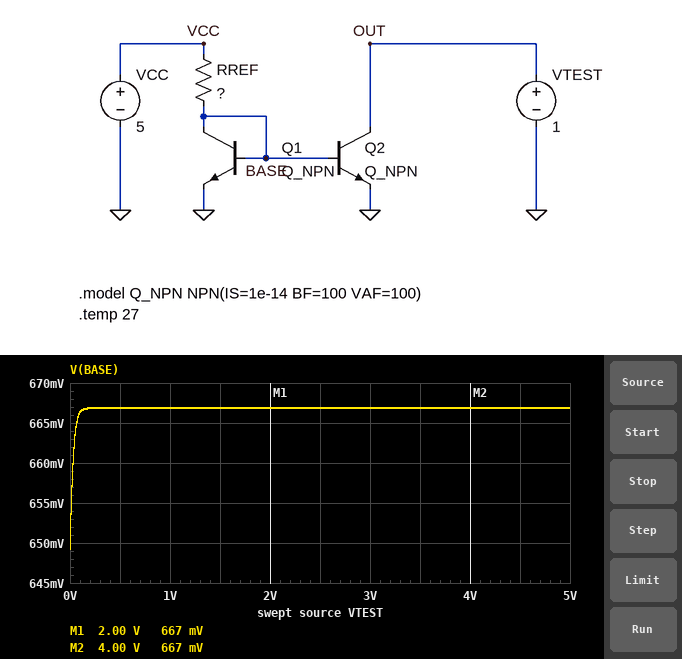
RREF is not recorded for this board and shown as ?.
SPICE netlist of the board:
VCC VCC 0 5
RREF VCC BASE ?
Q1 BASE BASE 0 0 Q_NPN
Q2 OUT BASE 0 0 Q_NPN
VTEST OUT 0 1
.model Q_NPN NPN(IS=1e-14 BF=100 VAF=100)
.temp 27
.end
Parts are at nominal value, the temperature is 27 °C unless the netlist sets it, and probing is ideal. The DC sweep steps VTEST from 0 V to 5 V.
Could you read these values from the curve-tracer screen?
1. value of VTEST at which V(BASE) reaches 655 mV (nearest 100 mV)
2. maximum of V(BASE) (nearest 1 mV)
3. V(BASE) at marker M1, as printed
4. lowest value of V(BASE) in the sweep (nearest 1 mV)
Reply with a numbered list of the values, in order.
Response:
1. 0 V
2. 667 mV
3. 667 mV
4. 649 mV
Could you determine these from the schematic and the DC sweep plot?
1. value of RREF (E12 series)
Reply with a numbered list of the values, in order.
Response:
1. 2.7 kΩ
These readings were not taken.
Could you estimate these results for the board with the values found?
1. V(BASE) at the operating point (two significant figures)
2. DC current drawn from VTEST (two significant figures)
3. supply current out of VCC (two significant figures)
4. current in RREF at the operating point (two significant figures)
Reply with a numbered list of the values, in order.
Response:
1. 670 mV
2. 1.6 mA
3. 1.6 mA
4. 1.6 mA
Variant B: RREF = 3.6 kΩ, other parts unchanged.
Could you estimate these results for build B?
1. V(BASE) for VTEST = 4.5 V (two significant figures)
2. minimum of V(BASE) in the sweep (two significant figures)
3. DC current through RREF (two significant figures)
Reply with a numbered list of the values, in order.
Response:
1. 660 mV
2. 640 mV
3. 1.2 mA
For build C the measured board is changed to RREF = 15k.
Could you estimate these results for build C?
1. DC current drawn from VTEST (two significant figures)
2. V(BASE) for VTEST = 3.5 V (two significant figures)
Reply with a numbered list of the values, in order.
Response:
1. 290 µA
2. 620 mV
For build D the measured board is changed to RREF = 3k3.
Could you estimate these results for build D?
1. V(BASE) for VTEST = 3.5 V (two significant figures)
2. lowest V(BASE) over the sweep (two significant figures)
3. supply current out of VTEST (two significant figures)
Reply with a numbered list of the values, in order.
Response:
1. 660 mV
2. 640 mV
3. 1.3 mA
